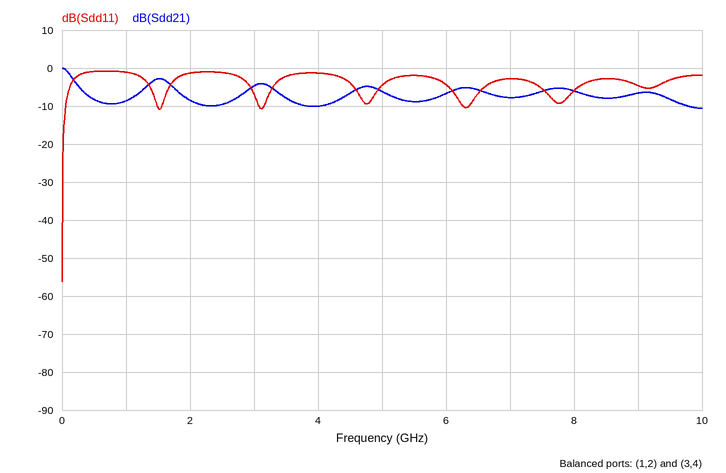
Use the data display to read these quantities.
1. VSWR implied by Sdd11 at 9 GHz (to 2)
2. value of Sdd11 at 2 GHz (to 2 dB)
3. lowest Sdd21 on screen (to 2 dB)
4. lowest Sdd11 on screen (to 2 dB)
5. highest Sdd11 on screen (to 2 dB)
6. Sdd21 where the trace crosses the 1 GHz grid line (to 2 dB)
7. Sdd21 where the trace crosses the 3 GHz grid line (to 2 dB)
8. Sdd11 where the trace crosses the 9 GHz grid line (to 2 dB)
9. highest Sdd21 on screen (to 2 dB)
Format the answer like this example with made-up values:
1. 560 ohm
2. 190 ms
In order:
1. 4
2. -2 dB
3. -10 dB
4. -56 dB
5. 0 dB
6. -8 dB
7. -4 dB
8. -4 dB
9. 0 dB
